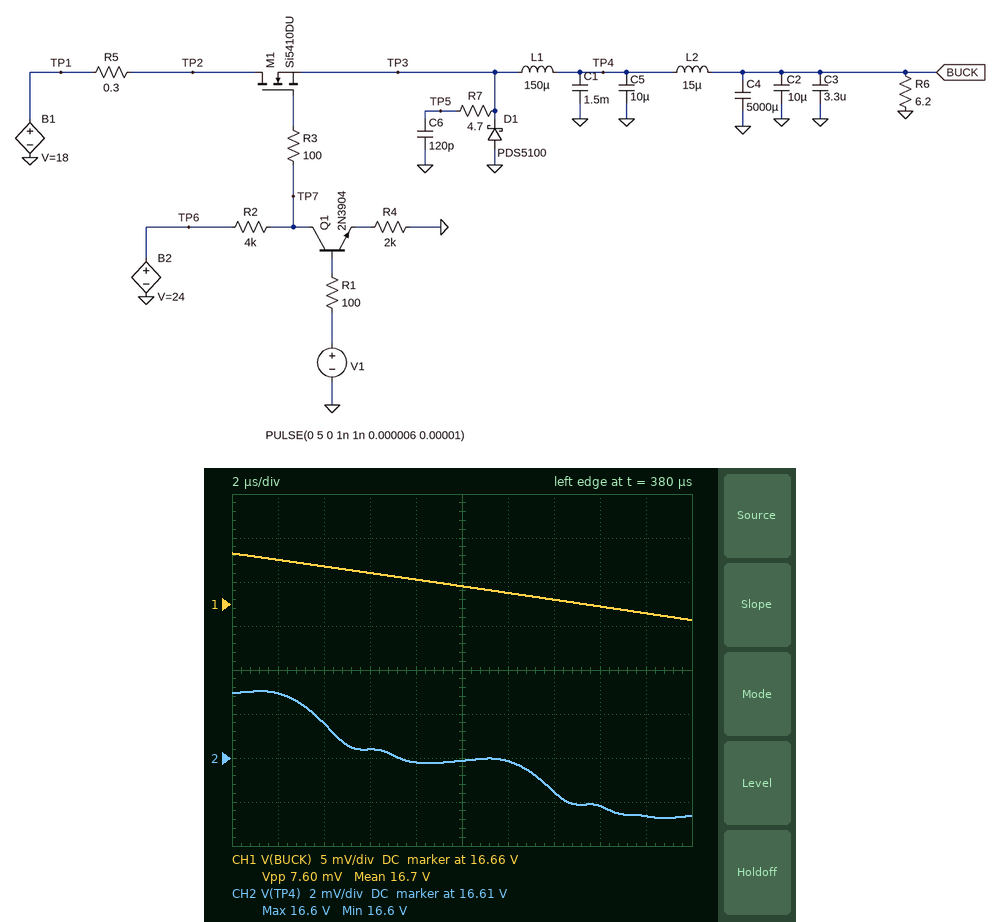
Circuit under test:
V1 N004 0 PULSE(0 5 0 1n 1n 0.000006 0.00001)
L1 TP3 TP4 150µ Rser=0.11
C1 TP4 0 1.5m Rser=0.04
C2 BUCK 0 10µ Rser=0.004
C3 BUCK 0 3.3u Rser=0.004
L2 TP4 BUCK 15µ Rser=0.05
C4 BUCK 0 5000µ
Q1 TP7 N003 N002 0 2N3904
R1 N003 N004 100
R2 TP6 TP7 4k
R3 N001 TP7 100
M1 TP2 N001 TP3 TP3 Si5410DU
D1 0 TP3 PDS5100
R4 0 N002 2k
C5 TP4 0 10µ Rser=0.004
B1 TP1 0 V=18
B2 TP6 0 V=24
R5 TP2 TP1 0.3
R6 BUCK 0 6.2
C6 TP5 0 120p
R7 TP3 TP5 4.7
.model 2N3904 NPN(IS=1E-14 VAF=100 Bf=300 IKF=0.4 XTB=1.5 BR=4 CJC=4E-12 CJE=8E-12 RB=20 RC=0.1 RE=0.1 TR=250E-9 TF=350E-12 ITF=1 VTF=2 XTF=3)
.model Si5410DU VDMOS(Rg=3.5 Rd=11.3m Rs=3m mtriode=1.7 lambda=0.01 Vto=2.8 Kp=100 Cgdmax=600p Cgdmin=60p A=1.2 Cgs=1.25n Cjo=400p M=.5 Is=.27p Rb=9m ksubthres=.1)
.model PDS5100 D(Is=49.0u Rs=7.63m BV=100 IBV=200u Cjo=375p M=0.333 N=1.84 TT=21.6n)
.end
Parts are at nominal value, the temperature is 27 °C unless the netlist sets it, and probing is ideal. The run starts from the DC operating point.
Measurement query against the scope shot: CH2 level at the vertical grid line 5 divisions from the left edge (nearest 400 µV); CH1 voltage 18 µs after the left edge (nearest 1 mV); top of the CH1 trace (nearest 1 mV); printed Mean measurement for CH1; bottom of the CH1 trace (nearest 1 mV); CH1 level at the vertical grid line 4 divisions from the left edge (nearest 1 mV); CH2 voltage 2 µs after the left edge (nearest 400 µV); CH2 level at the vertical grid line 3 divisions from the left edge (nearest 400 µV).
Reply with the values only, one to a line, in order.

16.6080 V
16.659 V
16.666 V
16.7 V
16.658 V
16.663 V
16.6108 V
16.6084 V
